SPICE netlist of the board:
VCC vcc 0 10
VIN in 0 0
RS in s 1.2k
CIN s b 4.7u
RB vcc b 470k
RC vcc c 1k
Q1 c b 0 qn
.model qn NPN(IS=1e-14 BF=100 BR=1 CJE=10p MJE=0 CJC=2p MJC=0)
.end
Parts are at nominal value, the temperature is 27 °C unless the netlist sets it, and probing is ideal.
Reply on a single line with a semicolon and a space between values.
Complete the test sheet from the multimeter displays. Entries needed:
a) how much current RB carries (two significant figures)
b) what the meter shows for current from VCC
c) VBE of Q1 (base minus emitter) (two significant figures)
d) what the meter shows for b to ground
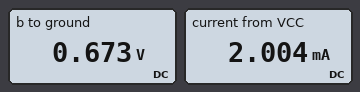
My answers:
20 µA; 2.004 mA; 670 mV; 0.673 V
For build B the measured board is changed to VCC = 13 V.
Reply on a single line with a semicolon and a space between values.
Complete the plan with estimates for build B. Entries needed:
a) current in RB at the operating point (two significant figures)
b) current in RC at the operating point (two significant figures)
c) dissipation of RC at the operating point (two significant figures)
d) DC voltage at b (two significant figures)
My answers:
26 µA; 2.6 mA; 6.9 mW; 680 mV
